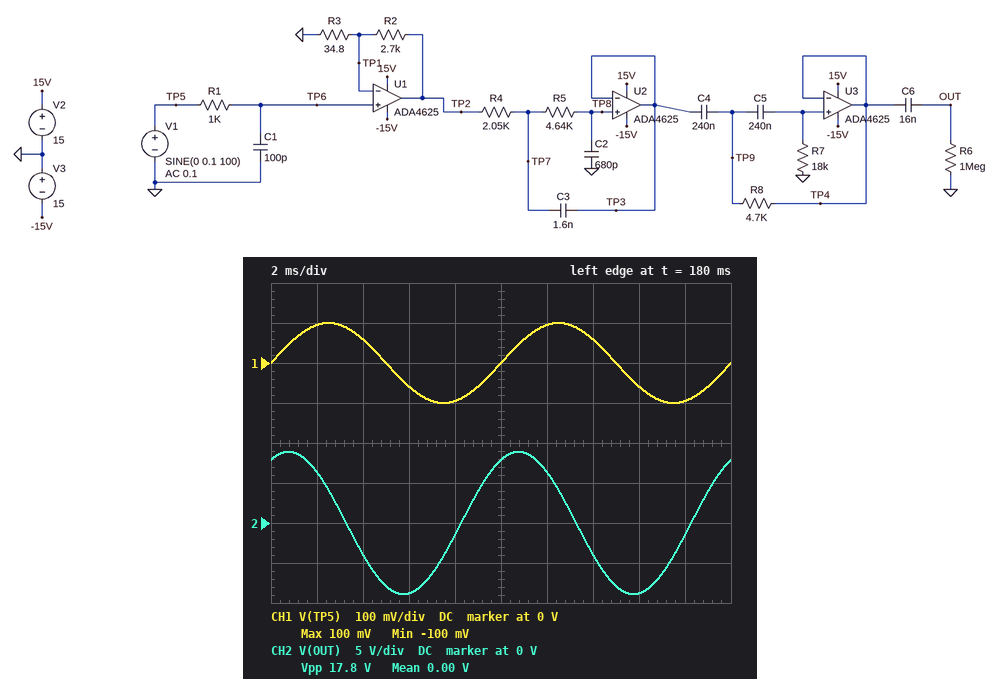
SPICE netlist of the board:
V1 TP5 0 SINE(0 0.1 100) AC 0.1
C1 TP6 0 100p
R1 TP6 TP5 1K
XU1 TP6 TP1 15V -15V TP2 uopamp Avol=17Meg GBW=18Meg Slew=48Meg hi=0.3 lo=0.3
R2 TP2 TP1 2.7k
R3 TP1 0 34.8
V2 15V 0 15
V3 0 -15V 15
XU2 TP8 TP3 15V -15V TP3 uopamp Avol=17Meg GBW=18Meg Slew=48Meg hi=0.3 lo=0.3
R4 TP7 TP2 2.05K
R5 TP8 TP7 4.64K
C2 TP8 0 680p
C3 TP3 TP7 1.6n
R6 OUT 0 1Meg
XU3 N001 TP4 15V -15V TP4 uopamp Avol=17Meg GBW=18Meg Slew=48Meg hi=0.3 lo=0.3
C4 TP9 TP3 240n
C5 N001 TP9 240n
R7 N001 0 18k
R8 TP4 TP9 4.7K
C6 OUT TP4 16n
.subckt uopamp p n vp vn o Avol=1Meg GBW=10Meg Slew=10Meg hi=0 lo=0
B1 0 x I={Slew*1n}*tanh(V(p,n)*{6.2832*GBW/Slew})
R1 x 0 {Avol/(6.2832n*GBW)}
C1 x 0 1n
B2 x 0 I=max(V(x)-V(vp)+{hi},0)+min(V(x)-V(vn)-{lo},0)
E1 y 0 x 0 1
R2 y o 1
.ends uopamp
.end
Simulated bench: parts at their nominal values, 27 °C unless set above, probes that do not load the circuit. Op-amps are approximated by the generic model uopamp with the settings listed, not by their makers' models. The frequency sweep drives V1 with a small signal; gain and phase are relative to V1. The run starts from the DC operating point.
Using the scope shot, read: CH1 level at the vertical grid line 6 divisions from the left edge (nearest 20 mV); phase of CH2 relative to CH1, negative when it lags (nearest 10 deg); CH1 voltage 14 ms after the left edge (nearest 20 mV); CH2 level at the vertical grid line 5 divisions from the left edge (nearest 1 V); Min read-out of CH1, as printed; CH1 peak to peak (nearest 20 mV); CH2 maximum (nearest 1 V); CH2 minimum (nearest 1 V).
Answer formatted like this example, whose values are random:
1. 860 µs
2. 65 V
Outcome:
1. 100 mV
2. 60 deg
3. 60 mV
4. 8 V
5. -100 mV
6. 200 mV
7. 9 V
8. -9 V
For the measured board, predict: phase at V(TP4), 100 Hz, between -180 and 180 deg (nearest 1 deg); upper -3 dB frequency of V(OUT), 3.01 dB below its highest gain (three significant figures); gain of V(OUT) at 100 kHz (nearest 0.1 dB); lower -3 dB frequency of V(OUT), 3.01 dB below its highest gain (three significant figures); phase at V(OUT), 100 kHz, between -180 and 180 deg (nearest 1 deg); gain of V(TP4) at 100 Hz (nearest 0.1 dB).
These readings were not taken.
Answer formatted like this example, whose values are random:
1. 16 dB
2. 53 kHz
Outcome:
1. 57 deg
2. 41.8 kHz
3. 24.6 dB
4. 62.2 Hz
5. -165 deg
6. 39.0 dB
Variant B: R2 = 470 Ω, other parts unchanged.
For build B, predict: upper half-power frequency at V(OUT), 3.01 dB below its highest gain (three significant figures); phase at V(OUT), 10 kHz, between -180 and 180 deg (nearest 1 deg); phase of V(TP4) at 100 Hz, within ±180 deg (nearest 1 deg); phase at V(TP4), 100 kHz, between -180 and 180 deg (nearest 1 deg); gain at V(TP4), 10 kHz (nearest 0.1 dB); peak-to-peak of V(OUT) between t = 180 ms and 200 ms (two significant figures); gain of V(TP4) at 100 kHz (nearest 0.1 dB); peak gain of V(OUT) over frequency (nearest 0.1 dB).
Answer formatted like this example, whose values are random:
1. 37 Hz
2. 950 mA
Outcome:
1. 42.7 kHz
2. -17 deg
3. 57 deg
4. -146 deg
5. 23.2 dB
6. 3.3 V
7. 10.7 dB
8. 24.3 dB
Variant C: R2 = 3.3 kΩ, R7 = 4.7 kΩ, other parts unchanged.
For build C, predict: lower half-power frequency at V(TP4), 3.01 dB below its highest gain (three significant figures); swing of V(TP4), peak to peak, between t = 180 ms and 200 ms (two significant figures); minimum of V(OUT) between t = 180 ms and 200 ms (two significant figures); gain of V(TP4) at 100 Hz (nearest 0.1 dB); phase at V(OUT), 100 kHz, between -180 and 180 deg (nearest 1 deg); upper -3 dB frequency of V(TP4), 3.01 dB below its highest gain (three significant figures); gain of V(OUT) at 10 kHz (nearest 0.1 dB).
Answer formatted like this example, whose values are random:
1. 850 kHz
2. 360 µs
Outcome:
1. 219 Hz
2. 6.4 V
3. -3.2 V
4. 30.1 dB
5. -169 deg
6. 47.9 kHz
7. 39.6 dB
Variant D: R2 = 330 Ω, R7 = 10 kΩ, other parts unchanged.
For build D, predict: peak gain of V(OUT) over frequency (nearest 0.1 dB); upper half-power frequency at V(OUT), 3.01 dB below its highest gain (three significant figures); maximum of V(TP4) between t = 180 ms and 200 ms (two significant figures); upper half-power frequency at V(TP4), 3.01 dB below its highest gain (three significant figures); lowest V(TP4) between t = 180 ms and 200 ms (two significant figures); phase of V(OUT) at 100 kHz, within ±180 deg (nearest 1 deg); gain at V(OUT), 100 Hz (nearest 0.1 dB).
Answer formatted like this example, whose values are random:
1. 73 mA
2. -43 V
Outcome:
1. 20.4 dB
2. 49.4 kHz
3. 790 mV
4. 49.3 kHz
5. -790 mV
6. -145 deg
7. 17.9 dB
